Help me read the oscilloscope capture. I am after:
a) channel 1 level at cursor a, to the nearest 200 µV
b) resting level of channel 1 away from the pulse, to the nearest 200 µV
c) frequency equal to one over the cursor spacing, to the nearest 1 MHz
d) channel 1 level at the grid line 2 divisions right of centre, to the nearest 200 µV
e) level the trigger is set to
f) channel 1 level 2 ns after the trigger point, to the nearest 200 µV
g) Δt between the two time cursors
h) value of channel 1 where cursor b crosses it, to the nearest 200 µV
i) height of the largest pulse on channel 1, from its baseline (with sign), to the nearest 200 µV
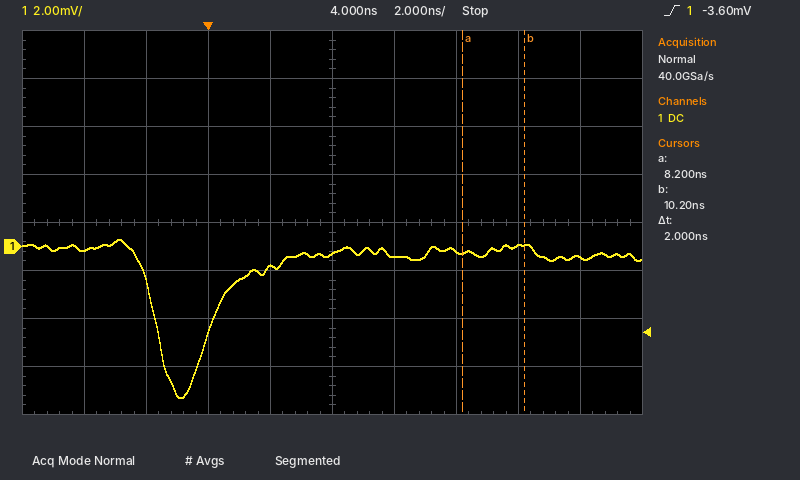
-200 µV
-400 µV
500 MHz
-200 µV
-3.60 mV
-800 µV
2 ns
0.0 mV
-6.0 mV
